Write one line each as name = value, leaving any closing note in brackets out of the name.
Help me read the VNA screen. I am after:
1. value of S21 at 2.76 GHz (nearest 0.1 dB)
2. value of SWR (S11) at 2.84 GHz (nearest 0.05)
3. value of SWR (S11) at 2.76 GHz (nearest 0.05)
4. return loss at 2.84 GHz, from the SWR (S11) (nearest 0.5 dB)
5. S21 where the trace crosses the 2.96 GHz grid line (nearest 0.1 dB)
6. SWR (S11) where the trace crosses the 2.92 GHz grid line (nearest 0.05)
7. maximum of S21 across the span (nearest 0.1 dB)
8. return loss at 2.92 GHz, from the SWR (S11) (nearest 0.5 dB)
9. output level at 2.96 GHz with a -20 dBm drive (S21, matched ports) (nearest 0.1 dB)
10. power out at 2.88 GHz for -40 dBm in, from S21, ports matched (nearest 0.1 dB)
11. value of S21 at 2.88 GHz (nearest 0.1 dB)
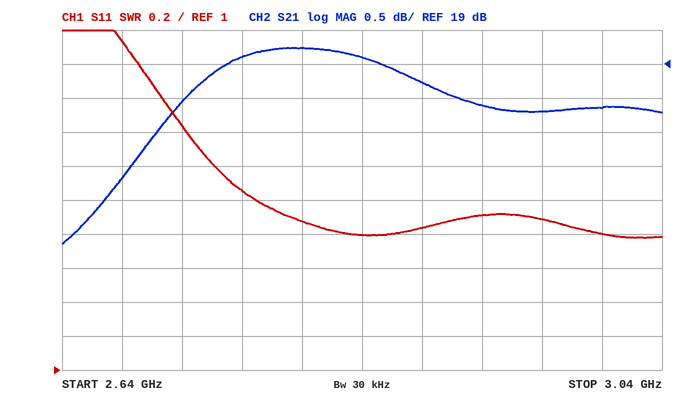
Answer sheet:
value of S21 at 2.76 GHz = 19.1 dB
value of SWR (S11) at 2.84 GHz = 1.80
value of SWR (S11) at 2.76 GHz = 2.05
return loss at 2.84 GHz, from the SWR (S11) = 11.0 dB
S21 where the trace crosses the 2.96 GHz grid line = 18.3 dB
SWR (S11) where the trace crosses the 2.92 GHz grid line = 1.90
maximum of S21 across the span = 19.2 dB
return loss at 2.92 GHz, from the SWR (S11) = 10.0 dB
output level at 2.96 GHz with a -20 dBm drive (S21, matched ports) = -1.7 dBm
power out at 2.88 GHz for -40 dBm in, from S21, ports matched = -21.3 dBm
value of S21 at 2.88 GHz = 18.7 dB
